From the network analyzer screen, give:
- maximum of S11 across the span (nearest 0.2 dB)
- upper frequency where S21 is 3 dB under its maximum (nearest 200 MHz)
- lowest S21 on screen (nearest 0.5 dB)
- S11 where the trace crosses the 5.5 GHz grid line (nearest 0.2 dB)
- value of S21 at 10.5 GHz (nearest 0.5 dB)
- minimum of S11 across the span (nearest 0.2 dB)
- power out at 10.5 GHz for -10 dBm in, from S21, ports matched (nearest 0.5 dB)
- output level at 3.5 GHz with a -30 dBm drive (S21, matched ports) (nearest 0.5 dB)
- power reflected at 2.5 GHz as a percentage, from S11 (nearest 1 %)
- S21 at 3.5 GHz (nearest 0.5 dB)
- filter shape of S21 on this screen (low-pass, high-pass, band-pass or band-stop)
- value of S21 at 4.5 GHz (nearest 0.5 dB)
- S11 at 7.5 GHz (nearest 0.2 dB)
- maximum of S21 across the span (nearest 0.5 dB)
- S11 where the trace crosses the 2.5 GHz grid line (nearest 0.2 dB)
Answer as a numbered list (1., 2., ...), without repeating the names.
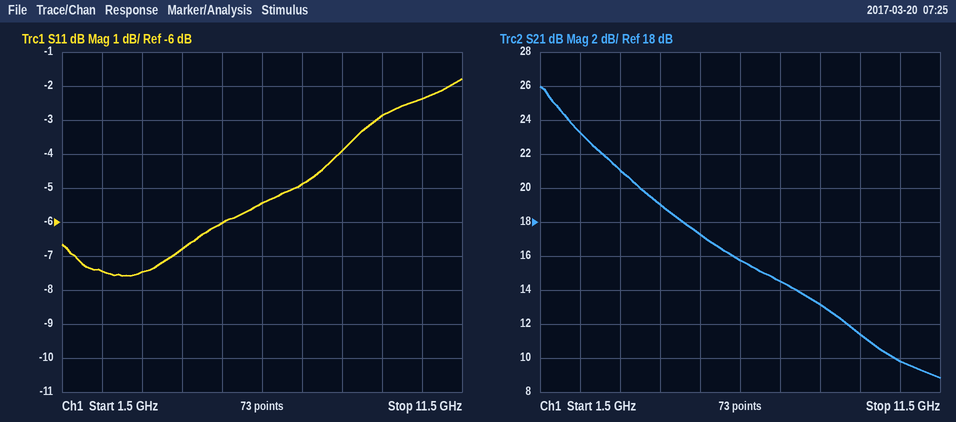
1. -1.8 dB
2. 2.6 GHz
3. 9.0 dB
4. -6.0 dB
5. 10.0 dB
6. -7.6 dB
7. 0.0 dBm
8. -9.0 dBm
9. 18 %
10. 21.0 dB
11. low-pass
12. 19.0 dB
13. -4.8 dB
14. 26.0 dB
15. -7.4 dB
